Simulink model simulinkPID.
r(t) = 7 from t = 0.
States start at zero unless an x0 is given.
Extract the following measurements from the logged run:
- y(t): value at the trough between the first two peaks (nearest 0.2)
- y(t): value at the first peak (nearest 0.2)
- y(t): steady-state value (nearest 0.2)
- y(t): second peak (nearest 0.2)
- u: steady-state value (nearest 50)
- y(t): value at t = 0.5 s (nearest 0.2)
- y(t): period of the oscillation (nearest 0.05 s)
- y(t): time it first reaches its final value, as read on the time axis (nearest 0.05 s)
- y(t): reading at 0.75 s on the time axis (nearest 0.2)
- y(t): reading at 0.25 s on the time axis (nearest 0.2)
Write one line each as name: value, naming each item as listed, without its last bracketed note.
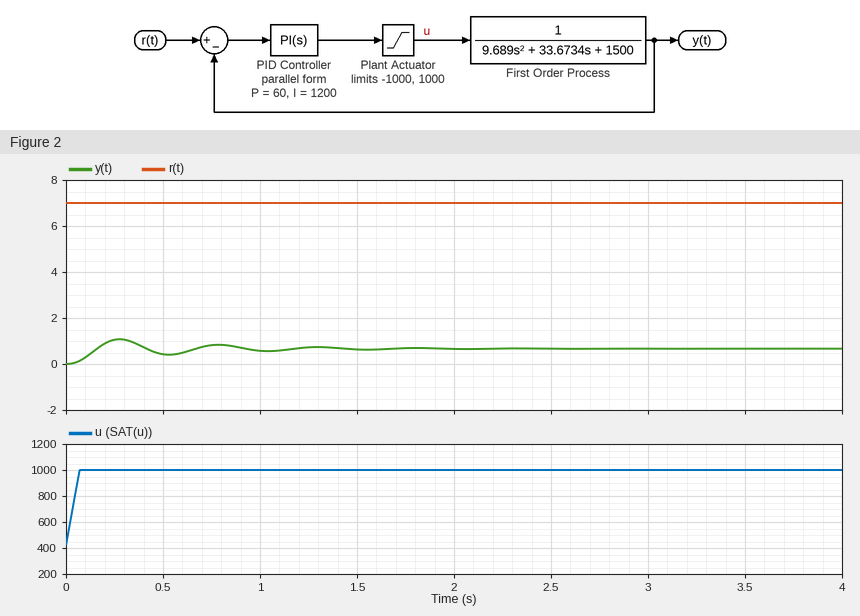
y(t): value at the trough between the first two peaks: 0.4
y(t): value at the first peak: 1.0
y(t): steady-state value: 0.6
y(t): second peak: 0.8
u: steady-state value: 1000
y(t): value at t = 0.5 s: 0.4
y(t): period of the oscillation: 0.50 s
y(t): time it first reaches its final value, as read on the time axis: 0.15 s
y(t): reading at 0.75 s on the time axis: 0.8
y(t): reading at 0.25 s on the time axis: 1.0
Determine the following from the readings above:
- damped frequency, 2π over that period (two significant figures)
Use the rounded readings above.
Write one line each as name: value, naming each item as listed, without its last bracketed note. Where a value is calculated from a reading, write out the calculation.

damped frequency, 2π over that period: 2π / 0.5 = 13 rad/s
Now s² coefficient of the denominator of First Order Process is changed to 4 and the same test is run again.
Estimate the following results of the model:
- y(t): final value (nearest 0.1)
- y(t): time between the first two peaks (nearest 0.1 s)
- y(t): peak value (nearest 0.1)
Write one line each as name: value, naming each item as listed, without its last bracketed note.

y(t): final value: 0.7
y(t): time between the first two peaks: 0.3 s
y(t): peak value: 1.0
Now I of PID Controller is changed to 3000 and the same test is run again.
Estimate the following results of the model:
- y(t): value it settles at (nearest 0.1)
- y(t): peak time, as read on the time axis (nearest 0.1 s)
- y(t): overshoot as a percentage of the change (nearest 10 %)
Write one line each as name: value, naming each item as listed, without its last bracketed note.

y(t): value it settles at: 0.7
y(t): peak time, as read on the time axis: 0.3 s
y(t): overshoot as a percentage of the change: 60 %
